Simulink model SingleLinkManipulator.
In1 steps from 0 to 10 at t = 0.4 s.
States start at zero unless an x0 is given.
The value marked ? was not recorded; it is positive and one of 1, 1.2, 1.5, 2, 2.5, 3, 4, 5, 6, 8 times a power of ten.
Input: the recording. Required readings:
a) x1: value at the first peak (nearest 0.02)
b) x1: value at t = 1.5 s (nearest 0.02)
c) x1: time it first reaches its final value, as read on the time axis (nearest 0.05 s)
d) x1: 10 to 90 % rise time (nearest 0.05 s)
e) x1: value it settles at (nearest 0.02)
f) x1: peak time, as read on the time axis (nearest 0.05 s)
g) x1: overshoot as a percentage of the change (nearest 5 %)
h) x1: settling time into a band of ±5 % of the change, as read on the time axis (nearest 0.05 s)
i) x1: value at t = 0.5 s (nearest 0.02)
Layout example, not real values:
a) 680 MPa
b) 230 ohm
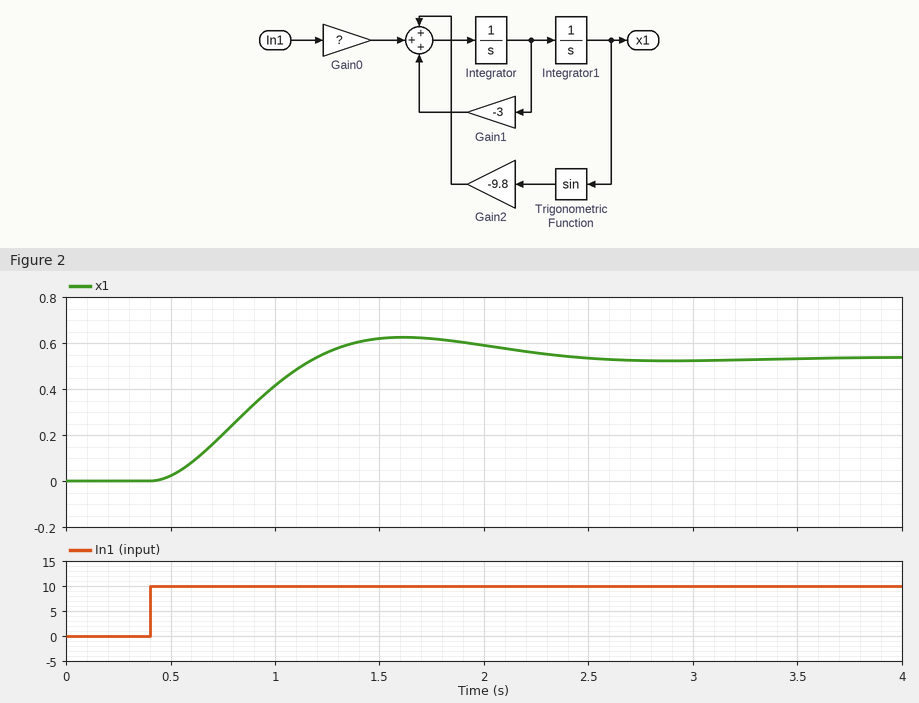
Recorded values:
a) 0.62
b) 0.62
c) 1.20 s
d) 0.55 s
e) 0.54
f) 1.60 s
g) 15 %
h) 2.20 s
i) 0.02
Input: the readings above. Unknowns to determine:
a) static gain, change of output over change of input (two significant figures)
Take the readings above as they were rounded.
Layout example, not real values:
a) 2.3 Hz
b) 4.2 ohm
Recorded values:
a) 0.054
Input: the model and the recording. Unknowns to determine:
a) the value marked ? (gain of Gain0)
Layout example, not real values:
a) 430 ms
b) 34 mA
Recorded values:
a) 0.5
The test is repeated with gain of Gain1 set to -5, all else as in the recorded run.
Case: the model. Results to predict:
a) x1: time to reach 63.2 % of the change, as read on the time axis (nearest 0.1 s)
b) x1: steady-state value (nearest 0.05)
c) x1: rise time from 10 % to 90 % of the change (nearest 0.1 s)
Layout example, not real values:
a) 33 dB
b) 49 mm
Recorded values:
a) 1.0 s
b) 0.55
c) 0.9 s
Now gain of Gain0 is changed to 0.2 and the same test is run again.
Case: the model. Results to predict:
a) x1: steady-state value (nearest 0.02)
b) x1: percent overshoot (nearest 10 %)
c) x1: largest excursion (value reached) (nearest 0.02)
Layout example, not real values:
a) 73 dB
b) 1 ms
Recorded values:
a) 0.20
b) 20 %
c) 0.24
